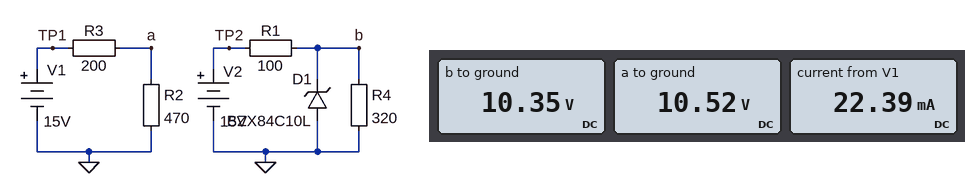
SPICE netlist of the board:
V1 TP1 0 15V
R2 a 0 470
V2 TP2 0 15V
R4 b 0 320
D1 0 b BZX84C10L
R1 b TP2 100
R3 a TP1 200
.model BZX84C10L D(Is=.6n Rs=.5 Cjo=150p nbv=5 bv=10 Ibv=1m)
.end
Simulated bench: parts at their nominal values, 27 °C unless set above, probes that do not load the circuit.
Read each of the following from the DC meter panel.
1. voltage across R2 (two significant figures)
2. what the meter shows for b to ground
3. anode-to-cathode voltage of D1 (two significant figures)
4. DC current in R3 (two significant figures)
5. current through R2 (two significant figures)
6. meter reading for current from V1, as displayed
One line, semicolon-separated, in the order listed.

11 V; 10.35 V; -10 V; 22 mA; 22 mA; 22.39 mA
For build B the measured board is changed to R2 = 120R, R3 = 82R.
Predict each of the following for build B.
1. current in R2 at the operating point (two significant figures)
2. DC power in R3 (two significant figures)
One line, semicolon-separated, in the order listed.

74 mA; 450 mW
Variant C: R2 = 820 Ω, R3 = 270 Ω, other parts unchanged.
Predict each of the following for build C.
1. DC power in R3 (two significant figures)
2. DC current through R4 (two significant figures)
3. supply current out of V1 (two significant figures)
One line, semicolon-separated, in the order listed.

51 mW; 32 mA; 14 mA
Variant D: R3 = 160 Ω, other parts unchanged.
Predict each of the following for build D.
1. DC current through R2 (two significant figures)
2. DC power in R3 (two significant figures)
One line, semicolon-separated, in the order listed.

24 mA; 91 mW
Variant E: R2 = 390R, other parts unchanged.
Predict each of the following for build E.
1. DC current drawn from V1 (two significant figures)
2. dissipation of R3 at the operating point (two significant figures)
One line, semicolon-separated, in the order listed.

25 mA; 130 mW
